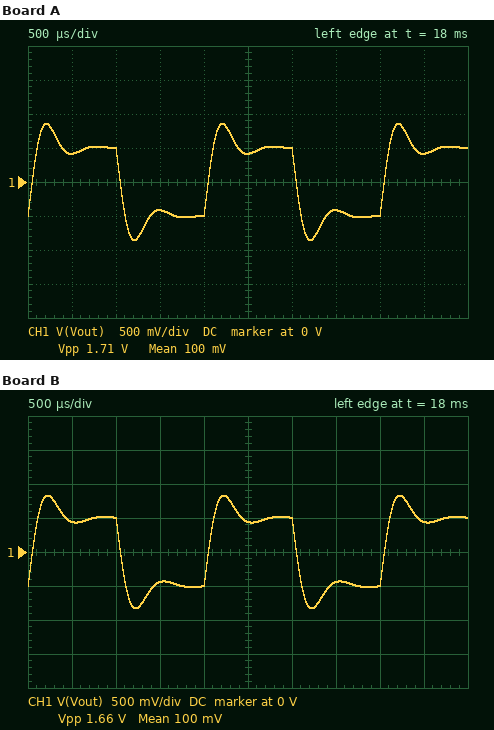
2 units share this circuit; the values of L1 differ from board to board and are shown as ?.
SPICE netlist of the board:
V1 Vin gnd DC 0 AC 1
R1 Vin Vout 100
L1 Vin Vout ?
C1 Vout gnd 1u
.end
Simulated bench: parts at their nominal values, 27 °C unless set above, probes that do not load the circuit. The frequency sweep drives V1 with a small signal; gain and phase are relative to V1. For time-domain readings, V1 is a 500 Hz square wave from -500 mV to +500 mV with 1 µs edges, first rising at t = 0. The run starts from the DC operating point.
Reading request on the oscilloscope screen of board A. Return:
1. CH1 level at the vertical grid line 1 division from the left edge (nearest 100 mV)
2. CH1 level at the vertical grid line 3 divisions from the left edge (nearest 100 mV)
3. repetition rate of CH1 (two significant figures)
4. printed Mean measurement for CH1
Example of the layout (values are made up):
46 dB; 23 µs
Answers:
400 mV; -400 mV; 500 Hz; 100 mV
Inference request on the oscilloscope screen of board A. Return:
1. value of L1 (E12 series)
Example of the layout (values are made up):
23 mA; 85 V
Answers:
6.8 mH
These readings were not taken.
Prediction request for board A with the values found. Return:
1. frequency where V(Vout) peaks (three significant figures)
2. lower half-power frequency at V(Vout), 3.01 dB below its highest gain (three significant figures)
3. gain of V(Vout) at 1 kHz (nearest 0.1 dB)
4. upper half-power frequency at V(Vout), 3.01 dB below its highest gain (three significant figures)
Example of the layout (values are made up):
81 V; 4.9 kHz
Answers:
1.71 kHz; 733 Hz; 2.2 dB; 2.51 kHz
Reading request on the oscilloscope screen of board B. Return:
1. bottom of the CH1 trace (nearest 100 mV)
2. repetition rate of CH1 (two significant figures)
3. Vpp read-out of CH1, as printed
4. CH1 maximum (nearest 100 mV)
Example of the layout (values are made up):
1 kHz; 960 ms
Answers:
-800 mV; 500 Hz; 1.66 V; 800 mV
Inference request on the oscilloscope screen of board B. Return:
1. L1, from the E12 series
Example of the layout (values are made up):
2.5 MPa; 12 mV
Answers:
8.2 mH
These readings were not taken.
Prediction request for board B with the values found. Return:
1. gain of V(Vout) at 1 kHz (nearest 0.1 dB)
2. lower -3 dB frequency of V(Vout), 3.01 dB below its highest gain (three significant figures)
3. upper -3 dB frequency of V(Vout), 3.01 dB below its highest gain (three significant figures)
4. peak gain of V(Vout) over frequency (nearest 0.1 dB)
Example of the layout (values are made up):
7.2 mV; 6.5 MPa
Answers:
2.4 dB; 529 Hz; 2.34 kHz; 3.8 dB
